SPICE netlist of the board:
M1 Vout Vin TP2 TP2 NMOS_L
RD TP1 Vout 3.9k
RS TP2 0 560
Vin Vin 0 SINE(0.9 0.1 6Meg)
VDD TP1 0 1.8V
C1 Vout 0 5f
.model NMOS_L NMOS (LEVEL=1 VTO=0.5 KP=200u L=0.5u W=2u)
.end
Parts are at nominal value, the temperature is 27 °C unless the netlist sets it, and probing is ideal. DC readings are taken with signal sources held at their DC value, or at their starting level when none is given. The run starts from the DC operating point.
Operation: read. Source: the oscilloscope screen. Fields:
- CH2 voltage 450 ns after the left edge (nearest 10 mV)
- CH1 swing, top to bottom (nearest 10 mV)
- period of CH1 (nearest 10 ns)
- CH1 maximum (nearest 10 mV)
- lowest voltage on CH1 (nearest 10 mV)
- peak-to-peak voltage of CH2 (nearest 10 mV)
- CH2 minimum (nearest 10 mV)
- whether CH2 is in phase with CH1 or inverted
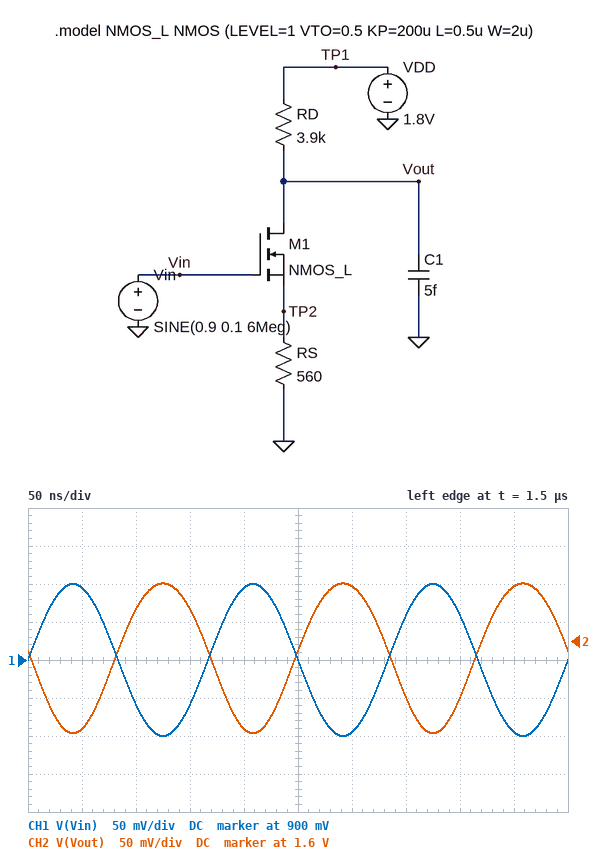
1.67 V
200 mV
170 ns
1.00 V
800 mV
200 mV
1.48 V
inverted
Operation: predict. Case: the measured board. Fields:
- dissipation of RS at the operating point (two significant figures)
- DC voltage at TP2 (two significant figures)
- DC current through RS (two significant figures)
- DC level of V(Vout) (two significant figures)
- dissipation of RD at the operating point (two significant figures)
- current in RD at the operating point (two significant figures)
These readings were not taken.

1.7 µW
31 mV
55 µA
1.6 V
12 µW
55 µA
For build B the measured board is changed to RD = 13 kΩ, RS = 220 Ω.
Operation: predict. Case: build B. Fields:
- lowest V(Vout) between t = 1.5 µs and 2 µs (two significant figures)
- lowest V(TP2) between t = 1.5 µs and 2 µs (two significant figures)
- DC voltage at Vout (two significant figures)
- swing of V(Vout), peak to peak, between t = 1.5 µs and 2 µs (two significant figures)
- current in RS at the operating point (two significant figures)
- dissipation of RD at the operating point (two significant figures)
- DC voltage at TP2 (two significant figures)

600 mV
7.5 mV
1.0 V
750 mV
60 µA
47 µW
13 mV
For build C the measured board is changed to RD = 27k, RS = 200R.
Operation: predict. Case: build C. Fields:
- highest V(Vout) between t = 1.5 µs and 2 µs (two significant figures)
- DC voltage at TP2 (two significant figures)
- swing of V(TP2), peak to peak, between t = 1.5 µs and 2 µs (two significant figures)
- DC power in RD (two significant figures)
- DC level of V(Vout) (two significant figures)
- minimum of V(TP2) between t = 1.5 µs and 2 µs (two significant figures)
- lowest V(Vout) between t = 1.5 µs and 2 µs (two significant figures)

870 mV
11 mV
5.0 mV
84 µW
290 mV
6.9 mV
200 mV
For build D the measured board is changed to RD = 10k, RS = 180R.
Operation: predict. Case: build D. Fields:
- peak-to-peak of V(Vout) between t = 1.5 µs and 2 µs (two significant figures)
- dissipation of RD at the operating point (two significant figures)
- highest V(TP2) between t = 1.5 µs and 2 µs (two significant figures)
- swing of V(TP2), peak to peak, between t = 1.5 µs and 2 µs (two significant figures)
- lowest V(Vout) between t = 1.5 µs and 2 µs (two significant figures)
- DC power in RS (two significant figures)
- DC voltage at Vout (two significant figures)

590 mV
37 µW
17 mV
11 mV
870 mV
660 nW
1.2 V
